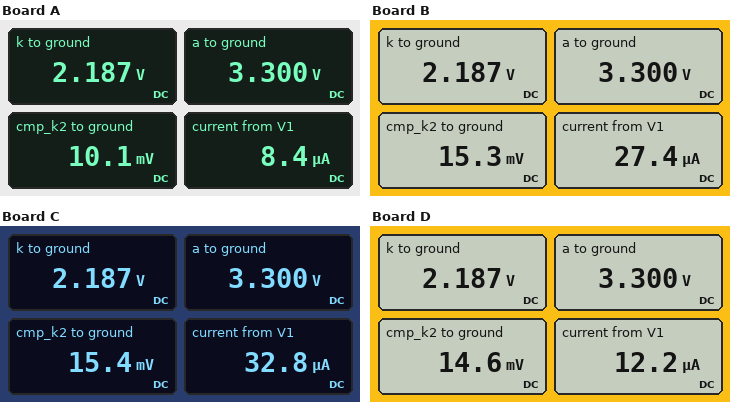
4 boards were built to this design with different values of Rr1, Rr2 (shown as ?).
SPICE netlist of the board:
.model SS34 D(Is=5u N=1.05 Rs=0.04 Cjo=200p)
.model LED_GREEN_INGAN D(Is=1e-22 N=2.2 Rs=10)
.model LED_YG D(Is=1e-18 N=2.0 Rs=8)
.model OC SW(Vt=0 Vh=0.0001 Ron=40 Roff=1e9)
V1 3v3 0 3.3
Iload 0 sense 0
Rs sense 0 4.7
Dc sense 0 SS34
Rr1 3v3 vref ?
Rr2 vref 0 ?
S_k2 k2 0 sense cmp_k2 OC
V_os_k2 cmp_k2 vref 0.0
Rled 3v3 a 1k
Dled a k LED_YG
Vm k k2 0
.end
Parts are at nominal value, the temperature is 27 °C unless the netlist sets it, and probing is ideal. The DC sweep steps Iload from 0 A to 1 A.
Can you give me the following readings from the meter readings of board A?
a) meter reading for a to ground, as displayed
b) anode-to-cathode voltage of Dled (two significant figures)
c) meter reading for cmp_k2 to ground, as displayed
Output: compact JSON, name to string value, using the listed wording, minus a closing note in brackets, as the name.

{"meter reading for a to ground, as displayed": "3.300 V", "anode-to-cathode voltage of Dled": "1.1 V", "meter reading for cmp_k2 to ground, as displayed": "10.1 mV"}
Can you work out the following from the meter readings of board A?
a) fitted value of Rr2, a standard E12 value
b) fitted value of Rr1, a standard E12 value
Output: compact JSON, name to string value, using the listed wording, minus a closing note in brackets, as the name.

{"fitted value of Rr2, a standard E12 value": "1.2 kΩ", "fitted value of Rr1, a standard E12 value": "390 kΩ"}
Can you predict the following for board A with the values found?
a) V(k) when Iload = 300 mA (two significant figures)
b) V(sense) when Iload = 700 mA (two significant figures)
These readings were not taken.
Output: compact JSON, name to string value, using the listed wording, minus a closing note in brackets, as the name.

{"V(k) when Iload = 300 mA": "57 mV", "V(sense) when Iload = 700 mA": "340 mV"}
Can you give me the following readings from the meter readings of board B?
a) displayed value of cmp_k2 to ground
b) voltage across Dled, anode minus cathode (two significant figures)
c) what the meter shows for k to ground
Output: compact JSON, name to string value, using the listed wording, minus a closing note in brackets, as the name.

{"displayed value of cmp_k2 to ground": "15.3 mV", "voltage across Dled, anode minus cathode": "1.1 V", "what the meter shows for k to ground": "2.187 V"}
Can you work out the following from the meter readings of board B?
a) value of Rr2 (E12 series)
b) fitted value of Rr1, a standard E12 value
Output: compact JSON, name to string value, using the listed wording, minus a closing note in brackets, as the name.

{"value of Rr2": "560 Ω", "fitted value of Rr1, a standard E12 value": "120 kΩ"}
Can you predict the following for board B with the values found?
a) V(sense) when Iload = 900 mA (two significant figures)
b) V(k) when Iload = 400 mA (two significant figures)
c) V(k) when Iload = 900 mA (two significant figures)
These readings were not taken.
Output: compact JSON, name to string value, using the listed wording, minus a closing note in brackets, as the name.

{"V(sense) when Iload = 900 mA": "360 mV", "V(k) when Iload = 400 mA": "57 mV", "V(k) when Iload = 900 mA": "57 mV"}
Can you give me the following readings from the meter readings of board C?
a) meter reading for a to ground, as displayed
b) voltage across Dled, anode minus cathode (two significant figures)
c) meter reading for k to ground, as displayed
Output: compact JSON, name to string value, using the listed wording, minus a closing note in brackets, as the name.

{"meter reading for a to ground, as displayed": "3.300 V", "voltage across Dled, anode minus cathode": "1.1 V", "meter reading for k to ground, as displayed": "2.187 V"}
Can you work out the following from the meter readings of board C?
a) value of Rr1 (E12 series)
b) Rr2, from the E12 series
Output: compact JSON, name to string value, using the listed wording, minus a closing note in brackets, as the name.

{"value of Rr1": "100 kΩ", "Rr2, from the E12 series": "470 Ω"}
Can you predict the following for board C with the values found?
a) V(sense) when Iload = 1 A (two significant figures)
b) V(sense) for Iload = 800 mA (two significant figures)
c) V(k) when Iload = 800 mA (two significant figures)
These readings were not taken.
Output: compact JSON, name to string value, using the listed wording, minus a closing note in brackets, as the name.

{"V(sense) when Iload = 1 A": "370 mV", "V(sense) for Iload = 800 mA": "350 mV", "V(k) when Iload = 800 mA": "57 mV"}
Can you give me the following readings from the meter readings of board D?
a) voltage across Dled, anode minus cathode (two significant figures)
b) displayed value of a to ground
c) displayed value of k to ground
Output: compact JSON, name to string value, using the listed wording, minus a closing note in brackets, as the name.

{"voltage across Dled, anode minus cathode": "1.1 V", "displayed value of a to ground": "3.300 V", "displayed value of k to ground": "2.187 V"}
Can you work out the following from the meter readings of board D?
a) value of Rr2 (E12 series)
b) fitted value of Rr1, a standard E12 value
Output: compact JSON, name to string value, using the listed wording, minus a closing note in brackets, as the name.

{"value of Rr2": "1.2 kΩ", "fitted value of Rr1, a standard E12 value": "270 kΩ"}
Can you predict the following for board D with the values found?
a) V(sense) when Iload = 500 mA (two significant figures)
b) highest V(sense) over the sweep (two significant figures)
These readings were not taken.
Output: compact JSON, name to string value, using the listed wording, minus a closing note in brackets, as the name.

{"V(sense) when Iload = 500 mA": "330 mV", "highest V(sense) over the sweep": "370 mV"}
